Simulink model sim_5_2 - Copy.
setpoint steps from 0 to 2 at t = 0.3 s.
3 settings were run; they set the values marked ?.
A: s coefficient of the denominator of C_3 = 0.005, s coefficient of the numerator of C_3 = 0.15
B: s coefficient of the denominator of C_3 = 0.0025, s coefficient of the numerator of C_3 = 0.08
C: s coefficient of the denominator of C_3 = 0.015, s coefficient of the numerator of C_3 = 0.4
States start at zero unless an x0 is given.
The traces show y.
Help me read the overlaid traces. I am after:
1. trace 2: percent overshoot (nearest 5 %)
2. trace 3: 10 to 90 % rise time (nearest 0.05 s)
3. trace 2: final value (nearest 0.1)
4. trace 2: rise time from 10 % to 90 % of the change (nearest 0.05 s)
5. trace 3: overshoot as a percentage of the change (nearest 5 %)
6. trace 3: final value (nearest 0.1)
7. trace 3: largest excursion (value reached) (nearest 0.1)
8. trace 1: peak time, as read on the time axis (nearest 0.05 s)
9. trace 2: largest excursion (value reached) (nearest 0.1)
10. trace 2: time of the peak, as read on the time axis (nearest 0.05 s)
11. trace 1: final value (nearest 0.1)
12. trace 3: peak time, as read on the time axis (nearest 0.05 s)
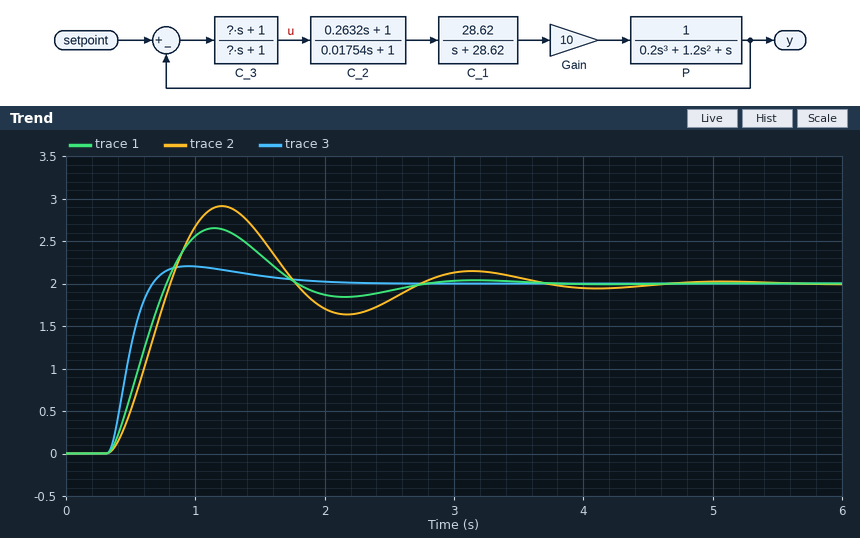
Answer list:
45 %
0.25 s
2.0
0.35 s
10 %
2.0
2.2
1.15 s
2.9
1.20 s
2.0
0.95 s
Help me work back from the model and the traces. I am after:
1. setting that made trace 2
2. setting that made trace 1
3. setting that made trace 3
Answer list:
B
A
C
